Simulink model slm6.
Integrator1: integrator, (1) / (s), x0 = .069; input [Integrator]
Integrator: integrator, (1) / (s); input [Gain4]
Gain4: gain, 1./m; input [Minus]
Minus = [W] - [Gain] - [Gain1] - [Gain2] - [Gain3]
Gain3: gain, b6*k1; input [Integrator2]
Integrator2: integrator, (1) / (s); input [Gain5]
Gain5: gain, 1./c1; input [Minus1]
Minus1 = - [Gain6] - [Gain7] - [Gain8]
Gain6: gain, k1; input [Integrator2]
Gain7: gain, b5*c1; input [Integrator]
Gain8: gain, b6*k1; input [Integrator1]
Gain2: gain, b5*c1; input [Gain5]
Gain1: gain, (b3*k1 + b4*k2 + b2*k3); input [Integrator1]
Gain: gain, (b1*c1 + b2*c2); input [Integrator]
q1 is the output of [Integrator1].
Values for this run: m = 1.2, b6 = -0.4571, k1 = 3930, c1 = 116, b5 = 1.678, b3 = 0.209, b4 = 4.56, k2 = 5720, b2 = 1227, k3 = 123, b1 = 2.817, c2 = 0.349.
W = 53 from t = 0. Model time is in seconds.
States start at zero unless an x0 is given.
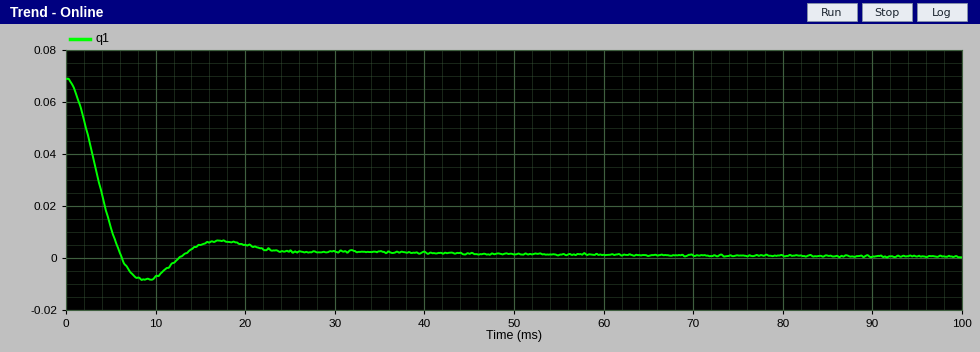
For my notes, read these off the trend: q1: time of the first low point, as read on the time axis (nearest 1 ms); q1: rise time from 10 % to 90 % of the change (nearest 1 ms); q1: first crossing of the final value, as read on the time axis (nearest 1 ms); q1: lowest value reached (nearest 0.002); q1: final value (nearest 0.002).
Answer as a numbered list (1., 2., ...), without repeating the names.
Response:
1. 9 ms
2. 4 ms
3. 6 ms
4. -0.008
5. 0.000
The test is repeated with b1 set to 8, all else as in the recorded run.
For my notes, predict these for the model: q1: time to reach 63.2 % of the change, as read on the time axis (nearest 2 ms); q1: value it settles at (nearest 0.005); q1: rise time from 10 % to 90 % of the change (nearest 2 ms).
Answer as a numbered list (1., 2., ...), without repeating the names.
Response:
1. 6 ms
2. 0.000
3. 12 ms
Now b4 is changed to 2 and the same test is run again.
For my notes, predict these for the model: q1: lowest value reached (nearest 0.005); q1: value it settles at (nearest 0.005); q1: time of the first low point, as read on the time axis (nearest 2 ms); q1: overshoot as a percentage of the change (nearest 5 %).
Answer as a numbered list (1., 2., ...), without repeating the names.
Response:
1. -0.005
2. 0.000
3. 10 ms
4. 10 %
